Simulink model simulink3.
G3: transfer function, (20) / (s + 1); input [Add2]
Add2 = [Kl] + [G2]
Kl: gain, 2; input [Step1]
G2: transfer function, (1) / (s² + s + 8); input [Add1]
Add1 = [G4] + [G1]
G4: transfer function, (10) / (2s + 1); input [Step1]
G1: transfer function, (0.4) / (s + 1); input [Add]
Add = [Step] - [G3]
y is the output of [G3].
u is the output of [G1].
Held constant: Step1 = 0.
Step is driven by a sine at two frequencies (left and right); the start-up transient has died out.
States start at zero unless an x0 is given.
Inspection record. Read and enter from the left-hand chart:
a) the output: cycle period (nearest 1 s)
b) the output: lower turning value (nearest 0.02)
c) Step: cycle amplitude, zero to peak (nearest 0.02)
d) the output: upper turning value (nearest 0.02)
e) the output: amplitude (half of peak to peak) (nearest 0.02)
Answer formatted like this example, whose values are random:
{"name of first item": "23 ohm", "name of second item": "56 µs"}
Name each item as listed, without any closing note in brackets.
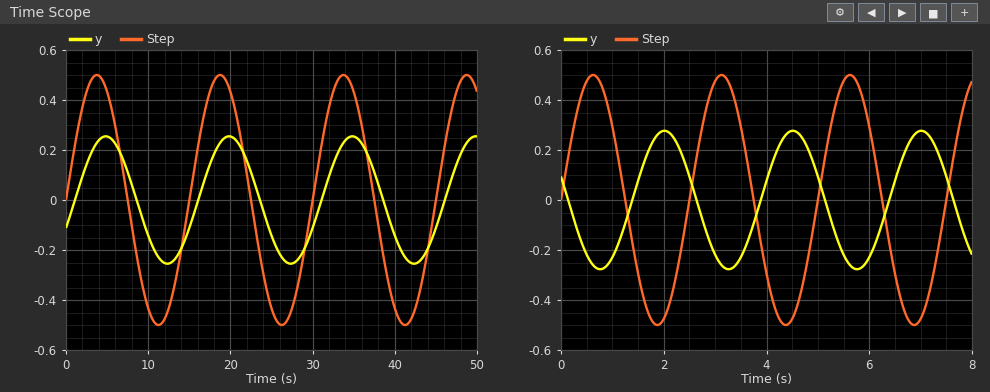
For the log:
{"the output: cycle period": "15 s", "the output: lower turning value": "-0.26", "Step: cycle amplitude, zero to peak": "0.50", "the output: upper turning value": "0.26", "the output: amplitude (half of peak to peak)": "0.26"}
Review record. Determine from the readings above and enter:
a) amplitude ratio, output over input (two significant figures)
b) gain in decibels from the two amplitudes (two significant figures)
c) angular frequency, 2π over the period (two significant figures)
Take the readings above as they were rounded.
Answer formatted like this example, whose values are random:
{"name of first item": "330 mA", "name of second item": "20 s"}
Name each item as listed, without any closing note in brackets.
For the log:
{"amplitude ratio, output over input": "0.52", "gain in decibels from the two amplitudes": "-5.7 dB", "angular frequency, 2π over the period": "0.42 rad/s"}
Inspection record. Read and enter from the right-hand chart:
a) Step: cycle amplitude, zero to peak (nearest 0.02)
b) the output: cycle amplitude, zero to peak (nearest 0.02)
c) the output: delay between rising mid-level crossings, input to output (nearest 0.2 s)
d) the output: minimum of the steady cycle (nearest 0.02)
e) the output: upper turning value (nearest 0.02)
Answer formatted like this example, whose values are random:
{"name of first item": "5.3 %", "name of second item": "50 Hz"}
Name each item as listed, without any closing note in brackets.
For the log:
{"Step: cycle amplitude, zero to peak": "0.50", "the output: cycle amplitude, zero to peak": "0.28", "the output: delay between rising mid-level crossings, input to output": "1.4 s", "the output: minimum of the steady cycle": "-0.28", "the output: upper turning value": "0.28"}
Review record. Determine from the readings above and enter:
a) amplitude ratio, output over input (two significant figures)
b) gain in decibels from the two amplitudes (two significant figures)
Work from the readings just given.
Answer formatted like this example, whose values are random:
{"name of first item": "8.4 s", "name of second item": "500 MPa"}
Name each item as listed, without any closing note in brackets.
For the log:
{"amplitude ratio, output over input": "0.56", "gain in decibels from the two amplitudes": "-5.0 dB"}
